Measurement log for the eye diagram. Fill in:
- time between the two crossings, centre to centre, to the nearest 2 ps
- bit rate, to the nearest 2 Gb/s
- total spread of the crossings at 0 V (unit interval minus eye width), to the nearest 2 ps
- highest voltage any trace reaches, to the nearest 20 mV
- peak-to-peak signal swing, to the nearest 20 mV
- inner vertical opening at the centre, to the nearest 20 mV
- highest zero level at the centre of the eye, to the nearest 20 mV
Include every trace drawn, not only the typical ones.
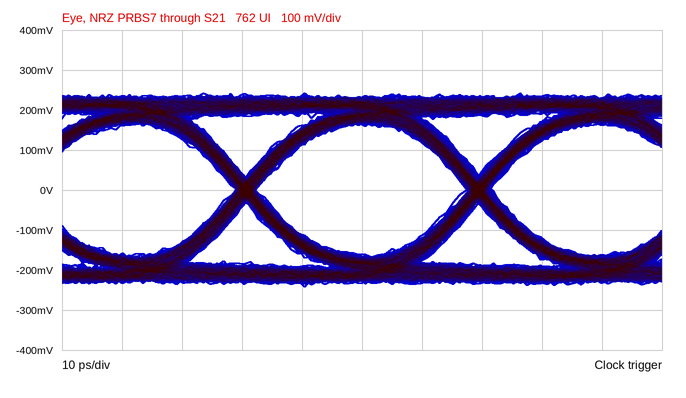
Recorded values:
38 ps
26 Gb/s
4 ps
240 mV
480 mV
320 mV
-160 mV
